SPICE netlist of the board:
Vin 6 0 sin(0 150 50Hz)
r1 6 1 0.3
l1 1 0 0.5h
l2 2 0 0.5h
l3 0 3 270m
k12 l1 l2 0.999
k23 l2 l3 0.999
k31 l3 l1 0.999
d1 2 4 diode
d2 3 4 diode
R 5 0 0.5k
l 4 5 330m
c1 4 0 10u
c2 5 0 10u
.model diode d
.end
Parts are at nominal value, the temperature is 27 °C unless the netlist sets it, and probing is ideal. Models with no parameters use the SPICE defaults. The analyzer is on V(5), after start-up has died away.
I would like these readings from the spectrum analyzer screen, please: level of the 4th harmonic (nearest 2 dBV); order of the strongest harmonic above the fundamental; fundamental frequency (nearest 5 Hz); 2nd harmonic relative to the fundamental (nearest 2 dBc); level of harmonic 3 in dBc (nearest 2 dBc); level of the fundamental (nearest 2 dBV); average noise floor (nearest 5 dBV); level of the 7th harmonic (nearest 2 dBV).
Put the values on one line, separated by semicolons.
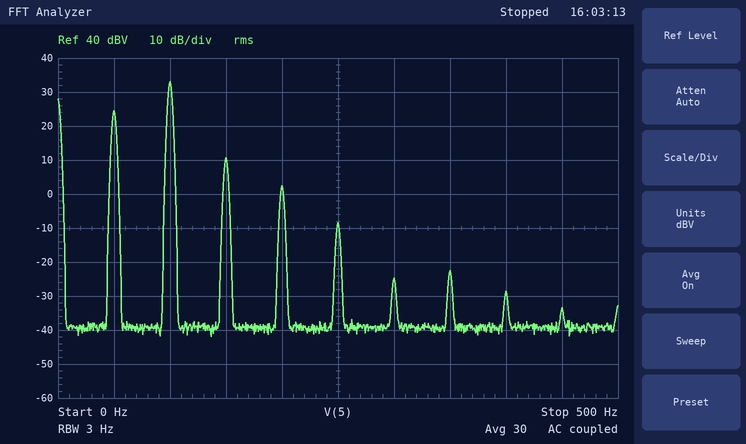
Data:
2 dBV; 2; 50 Hz; 8 dBc; -14 dBc; 24 dBV; -40 dBV; -22 dBV
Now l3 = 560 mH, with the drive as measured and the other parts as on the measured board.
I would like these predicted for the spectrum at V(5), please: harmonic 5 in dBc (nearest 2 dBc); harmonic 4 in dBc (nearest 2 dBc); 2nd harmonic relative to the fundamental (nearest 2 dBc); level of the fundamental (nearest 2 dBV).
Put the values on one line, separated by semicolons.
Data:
-30 dBc; -8 dBc; 22 dBc; 12 dBV
